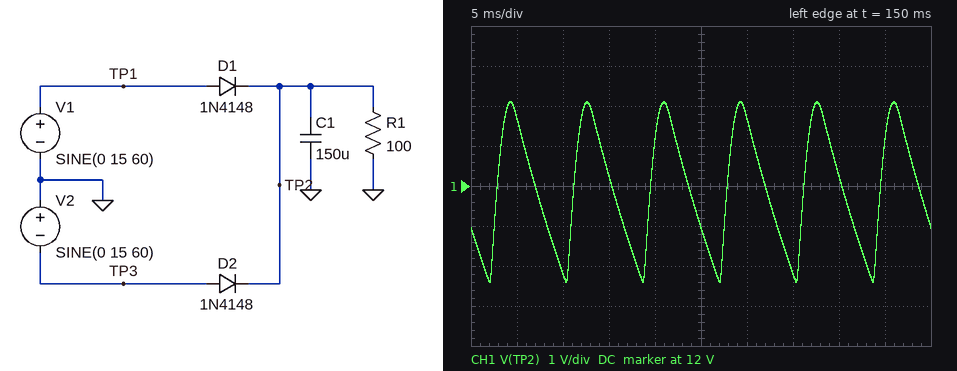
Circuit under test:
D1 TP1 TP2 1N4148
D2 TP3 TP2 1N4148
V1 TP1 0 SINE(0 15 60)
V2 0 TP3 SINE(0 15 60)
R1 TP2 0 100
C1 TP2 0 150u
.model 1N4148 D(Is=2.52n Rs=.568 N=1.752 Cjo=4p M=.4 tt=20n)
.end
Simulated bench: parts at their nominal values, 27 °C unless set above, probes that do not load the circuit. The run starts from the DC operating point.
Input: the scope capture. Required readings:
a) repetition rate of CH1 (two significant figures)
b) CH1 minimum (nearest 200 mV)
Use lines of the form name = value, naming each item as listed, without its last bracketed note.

repetition rate of CH1 = 120 Hz
CH1 minimum = 9.6 V
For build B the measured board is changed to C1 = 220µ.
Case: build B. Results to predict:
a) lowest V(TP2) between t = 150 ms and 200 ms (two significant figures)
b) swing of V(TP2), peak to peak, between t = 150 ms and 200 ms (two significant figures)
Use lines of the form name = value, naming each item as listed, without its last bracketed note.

lowest V(TP2) between t = 150 ms and 200 ms = 11 V
swing of V(TP2), peak to peak, between t = 150 ms and 200 ms = 3.4 V
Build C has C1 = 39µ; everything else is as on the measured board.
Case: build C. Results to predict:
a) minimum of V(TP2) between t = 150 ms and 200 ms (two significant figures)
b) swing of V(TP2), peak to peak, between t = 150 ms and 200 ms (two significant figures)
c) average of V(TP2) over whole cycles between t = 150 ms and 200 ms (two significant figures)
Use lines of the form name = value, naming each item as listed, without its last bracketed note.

minimum of V(TP2) between t = 150 ms and 200 ms = 4.7 V
swing of V(TP2), peak to peak, between t = 150 ms and 200 ms = 9.4 V
average of V(TP2) over whole cycles between t = 150 ms and 200 ms = 9.9 V
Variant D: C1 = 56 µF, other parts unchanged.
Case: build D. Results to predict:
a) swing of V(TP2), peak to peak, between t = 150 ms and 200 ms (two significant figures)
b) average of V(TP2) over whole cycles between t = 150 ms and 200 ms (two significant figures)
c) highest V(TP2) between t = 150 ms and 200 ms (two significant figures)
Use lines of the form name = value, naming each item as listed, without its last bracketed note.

swing of V(TP2), peak to peak, between t = 150 ms and 200 ms = 8.1 V
average of V(TP2) over whole cycles between t = 150 ms and 200 ms = 10 V
highest V(TP2) between t = 150 ms and 200 ms = 14 V
